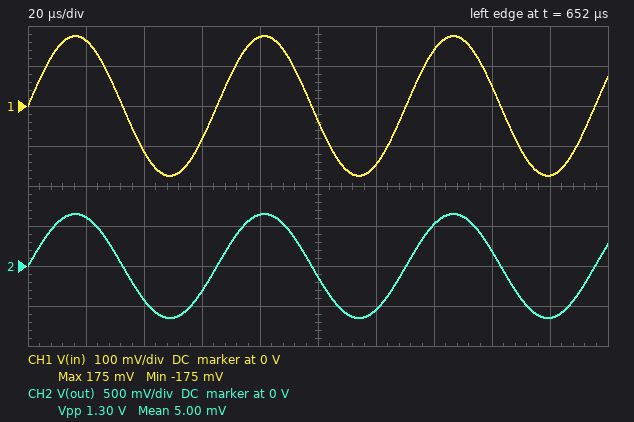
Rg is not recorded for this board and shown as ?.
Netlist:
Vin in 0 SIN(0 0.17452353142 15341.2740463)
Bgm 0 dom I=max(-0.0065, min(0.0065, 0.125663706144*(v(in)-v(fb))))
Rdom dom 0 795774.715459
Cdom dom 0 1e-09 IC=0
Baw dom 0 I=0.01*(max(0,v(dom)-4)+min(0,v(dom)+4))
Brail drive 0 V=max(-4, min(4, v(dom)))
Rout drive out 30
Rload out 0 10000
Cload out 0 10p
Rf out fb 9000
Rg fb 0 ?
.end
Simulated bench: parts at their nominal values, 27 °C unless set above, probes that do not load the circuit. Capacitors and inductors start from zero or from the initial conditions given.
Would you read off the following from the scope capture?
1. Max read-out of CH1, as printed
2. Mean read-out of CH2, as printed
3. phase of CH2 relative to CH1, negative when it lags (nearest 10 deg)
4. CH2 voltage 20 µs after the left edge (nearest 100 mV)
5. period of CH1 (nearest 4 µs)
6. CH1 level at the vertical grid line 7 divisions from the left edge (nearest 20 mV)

175 mV
5.00 mV
0 deg
600 mV
64 µs
140 mV
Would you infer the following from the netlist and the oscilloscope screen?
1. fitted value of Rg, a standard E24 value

3.3 kΩ
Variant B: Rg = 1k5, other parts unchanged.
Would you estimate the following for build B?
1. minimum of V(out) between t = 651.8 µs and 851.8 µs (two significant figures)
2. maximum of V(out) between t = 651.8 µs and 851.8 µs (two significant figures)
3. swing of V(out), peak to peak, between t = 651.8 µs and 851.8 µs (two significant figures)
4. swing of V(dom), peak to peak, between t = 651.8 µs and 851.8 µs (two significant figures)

-1.2 V
1.2 V
2.4 V
2.5 V
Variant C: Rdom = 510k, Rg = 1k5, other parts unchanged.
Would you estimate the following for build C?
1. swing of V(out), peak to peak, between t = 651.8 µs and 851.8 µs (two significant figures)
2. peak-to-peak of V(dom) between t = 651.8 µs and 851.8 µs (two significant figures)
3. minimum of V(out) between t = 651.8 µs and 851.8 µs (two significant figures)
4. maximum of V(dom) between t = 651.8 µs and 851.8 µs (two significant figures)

2.4 V
2.5 V
-1.2 V
1.2 V
